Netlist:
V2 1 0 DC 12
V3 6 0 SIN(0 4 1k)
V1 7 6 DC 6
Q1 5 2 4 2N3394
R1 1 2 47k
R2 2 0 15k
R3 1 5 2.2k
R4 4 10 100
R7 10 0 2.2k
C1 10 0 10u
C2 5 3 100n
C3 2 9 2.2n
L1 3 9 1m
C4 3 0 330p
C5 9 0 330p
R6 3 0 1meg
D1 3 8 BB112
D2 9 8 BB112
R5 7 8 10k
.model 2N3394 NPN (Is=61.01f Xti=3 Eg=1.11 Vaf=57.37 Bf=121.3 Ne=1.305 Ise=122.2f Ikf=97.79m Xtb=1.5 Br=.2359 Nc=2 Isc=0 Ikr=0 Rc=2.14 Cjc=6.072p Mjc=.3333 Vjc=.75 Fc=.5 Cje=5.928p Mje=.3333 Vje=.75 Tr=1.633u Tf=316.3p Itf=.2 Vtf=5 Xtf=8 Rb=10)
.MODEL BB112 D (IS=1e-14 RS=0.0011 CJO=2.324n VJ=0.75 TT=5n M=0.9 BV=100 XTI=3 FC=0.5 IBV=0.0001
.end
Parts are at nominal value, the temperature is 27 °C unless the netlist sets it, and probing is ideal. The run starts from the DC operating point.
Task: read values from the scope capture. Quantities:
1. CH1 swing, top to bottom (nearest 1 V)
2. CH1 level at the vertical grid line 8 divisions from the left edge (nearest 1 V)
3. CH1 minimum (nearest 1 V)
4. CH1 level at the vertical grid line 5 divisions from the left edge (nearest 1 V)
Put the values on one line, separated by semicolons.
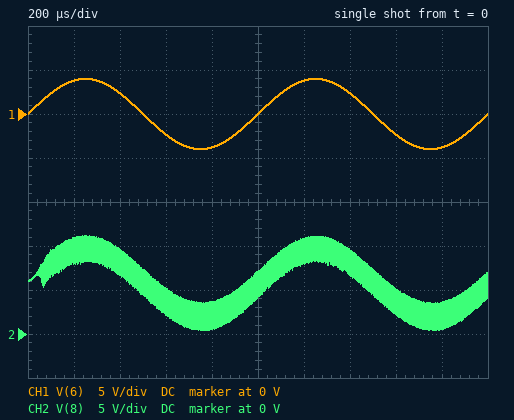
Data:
8 V; -2 V; -4 V; 0 V
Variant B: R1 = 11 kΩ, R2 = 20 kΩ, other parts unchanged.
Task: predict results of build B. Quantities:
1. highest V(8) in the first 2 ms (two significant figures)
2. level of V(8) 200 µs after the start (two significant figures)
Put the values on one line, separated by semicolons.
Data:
10 V; 9.8 V
